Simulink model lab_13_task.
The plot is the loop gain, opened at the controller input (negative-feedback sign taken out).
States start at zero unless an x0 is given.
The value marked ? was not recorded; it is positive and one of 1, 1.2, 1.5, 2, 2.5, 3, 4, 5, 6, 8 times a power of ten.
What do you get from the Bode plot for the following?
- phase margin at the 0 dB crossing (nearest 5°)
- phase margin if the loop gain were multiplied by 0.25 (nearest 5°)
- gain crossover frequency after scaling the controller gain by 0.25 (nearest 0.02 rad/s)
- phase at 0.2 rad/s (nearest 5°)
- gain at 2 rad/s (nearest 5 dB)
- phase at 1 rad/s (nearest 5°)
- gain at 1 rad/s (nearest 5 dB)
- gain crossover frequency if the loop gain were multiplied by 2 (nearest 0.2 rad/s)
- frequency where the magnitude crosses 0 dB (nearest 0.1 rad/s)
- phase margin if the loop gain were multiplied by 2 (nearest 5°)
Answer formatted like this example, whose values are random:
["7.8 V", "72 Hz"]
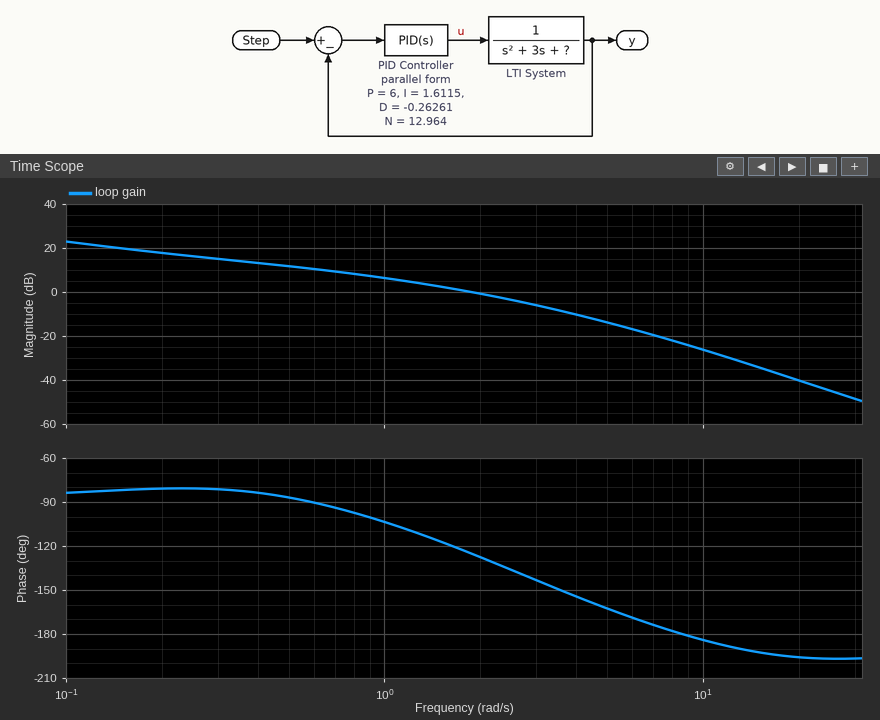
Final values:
["55°", "95°", "0.48 rad/s", "-80°", "0 dB", "-105°", "5 dB", "3.0 rad/s", "1.9 rad/s", "35°"]
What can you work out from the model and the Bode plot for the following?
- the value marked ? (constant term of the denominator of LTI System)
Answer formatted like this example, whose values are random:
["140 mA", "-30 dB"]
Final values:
["1.2"]
